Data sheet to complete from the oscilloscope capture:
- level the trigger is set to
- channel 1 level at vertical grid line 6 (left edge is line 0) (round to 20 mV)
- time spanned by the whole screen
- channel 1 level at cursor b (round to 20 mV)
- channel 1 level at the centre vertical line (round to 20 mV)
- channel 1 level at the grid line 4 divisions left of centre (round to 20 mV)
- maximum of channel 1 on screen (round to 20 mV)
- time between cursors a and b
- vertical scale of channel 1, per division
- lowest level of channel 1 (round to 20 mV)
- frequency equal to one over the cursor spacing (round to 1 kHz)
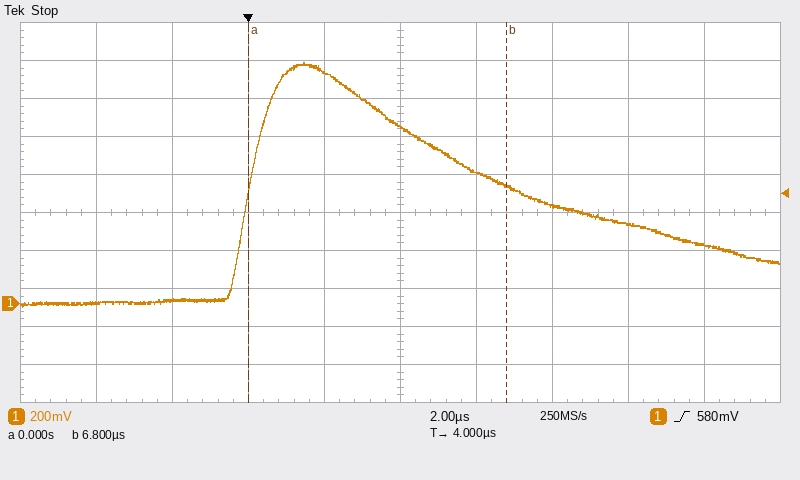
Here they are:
580 mV
700 mV
20 µs
620 mV
920 mV
0 mV
1.26 V
6.8 µs
200 mV
-20 mV
147 kHz
